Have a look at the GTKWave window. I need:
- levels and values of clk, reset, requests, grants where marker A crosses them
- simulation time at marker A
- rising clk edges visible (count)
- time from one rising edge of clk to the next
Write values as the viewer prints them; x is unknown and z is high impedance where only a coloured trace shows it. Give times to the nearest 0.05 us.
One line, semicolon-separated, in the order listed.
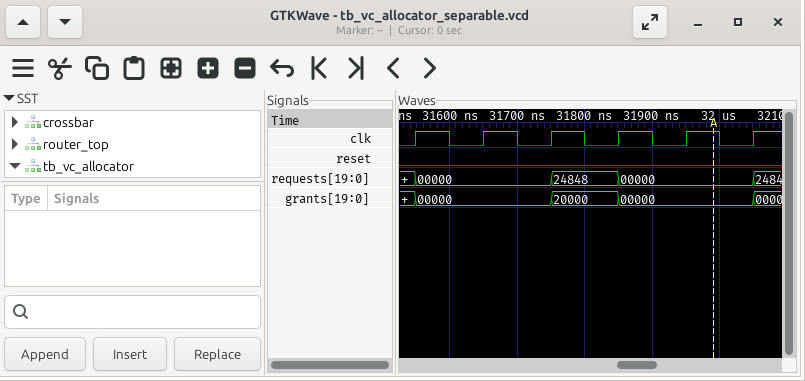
clk=1, reset=0, requests=00000, grants=00000; 32 us; 6; 0.1 us
